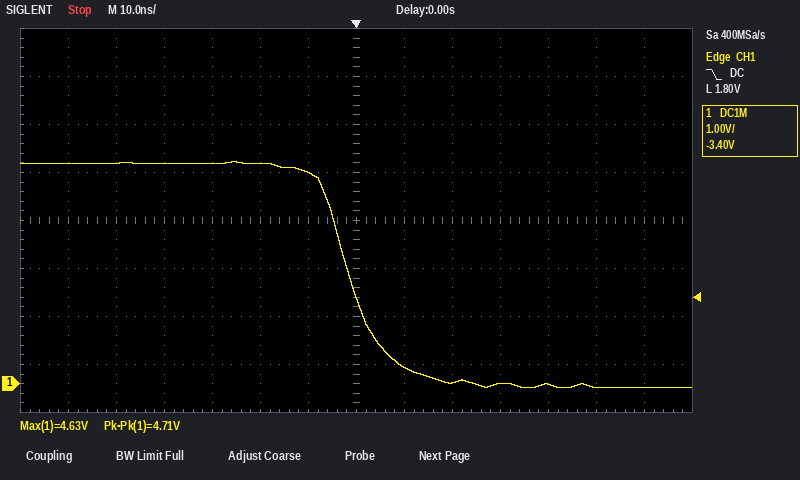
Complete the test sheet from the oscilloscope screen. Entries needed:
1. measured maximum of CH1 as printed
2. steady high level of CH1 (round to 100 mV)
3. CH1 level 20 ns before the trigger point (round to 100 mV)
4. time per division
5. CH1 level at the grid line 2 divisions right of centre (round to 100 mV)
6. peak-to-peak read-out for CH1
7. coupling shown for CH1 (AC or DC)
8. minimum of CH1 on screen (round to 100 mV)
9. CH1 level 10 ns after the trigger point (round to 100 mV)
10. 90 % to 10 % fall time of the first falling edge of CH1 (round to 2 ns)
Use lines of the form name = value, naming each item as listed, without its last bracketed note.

measured maximum of CH1 as printed = 4.63 V
steady high level of CH1 = 4.6 V
CH1 level 20 ns before the trigger point = 4.6 V
time per division = 10 ns
CH1 level at the grid line 2 divisions right of centre = 0.0 V
peak-to-peak read-out for CH1 = 4.71 V
coupling shown for CH1 = DC
minimum of CH1 on screen = -100 mV
CH1 level 10 ns after the trigger point = 300 mV
90 % to 10 % fall time of the first falling edge of CH1 = 16 ns
